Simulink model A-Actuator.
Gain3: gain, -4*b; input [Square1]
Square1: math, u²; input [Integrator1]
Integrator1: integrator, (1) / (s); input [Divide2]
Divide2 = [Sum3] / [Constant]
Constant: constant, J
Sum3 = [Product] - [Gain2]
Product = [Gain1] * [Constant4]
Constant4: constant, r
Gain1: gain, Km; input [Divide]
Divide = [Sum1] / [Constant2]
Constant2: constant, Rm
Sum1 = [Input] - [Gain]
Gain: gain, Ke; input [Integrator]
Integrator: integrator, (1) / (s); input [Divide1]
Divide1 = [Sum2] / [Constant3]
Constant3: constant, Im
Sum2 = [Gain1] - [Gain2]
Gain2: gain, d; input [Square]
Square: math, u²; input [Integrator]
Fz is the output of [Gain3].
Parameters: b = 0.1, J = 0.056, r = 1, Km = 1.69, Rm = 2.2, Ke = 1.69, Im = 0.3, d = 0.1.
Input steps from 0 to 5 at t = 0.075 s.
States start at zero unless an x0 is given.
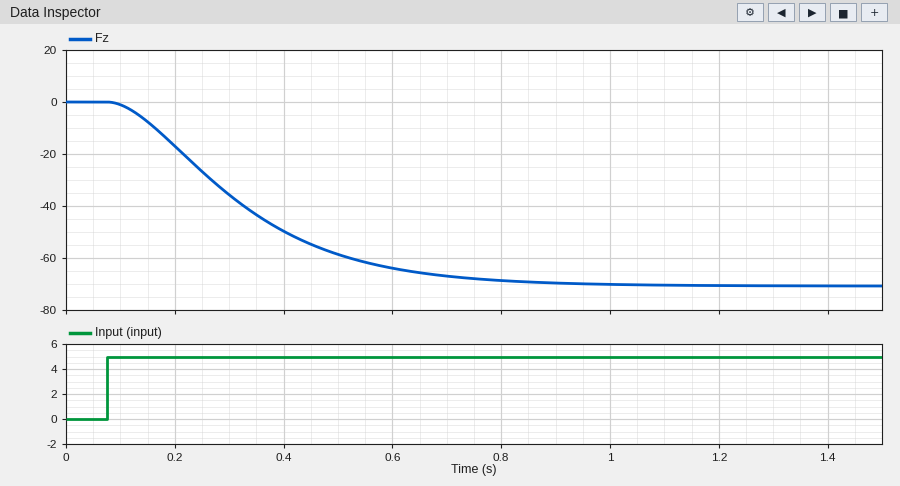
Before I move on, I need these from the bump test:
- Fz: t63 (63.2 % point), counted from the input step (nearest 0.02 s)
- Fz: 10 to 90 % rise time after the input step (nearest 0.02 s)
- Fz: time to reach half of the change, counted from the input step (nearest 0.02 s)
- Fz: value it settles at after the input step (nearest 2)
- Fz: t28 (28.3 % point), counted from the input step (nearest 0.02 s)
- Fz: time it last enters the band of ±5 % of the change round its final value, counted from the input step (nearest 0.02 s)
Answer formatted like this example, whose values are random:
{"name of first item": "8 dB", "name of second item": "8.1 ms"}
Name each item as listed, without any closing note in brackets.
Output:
{"Fz: t63 (63.2 % point), counted from the input step": "0.28 s", "Fz: 10 to 90 % rise time after the input step": "0.44 s", "Fz: time to reach half of the change, counted from the input step": "0.22 s", "Fz: value it settles at after the input step": "-70", "Fz: t28 (28.3 % point), counted from the input step": "0.14 s", "Fz: time it last enters the band of ±5 % of the change round its final value, counted from the input step": "0.64 s"}
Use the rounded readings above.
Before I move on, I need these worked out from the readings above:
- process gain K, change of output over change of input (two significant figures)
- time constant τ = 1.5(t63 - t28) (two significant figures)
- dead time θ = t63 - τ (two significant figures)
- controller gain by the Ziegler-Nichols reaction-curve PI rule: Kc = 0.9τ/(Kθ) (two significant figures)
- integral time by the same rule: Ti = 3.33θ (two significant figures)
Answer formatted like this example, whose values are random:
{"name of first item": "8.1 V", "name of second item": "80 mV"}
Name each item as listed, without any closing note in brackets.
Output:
{"process gain K, change of output over change of input": "-14", "time constant τ = 1.5(t63 - t28)": "0.21 s", "dead time θ = t63 - τ": "0.070 s", "controller gain by the Ziegler-Nichols reaction-curve PI rule: Kc = 0.9τ/(Kθ)": "-0.19", "integral time by the same rule: Ti = 3.33θ": "0.23 s"}
